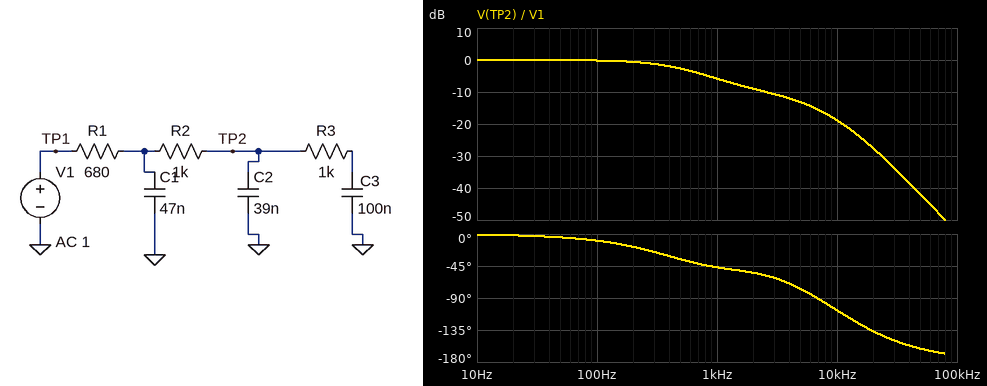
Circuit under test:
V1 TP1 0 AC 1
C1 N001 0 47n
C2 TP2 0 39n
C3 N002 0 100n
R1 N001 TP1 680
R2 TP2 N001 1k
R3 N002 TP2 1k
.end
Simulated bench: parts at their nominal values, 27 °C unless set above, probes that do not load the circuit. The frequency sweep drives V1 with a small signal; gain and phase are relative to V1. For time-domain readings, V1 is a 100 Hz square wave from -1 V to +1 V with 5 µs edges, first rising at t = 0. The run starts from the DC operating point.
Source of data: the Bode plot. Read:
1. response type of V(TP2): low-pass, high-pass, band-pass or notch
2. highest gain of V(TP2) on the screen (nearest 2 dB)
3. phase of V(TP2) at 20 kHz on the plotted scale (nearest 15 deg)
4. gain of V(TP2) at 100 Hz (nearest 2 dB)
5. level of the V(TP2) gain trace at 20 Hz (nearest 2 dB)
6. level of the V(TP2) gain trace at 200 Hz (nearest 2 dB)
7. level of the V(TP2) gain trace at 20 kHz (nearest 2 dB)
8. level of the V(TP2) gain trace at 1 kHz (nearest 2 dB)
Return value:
low-pass
0 dB
-135 deg
0 dB
0 dB
0 dB
-28 dB
-6 dB
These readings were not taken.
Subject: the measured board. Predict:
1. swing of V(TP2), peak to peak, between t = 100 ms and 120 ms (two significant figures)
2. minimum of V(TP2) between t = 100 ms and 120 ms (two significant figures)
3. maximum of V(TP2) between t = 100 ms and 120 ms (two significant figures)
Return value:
2.0 V
-1.0 V
1.0 V
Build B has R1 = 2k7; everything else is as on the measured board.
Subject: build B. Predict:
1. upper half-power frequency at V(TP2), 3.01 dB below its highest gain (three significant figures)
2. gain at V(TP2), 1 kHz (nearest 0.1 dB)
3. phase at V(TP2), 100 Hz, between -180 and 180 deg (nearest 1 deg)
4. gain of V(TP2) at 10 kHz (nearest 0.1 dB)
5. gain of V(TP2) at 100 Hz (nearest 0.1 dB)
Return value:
239 Hz
-11.8 dB
-22 deg
-29.6 dB
-0.7 dB
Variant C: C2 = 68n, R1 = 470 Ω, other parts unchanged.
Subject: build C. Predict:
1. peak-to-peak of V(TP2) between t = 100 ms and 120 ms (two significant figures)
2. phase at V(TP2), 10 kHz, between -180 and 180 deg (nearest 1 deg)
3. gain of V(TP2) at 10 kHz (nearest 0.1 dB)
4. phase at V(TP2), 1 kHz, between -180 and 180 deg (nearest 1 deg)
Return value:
2.0 V
-112 deg
-20.0 dB
-49 deg
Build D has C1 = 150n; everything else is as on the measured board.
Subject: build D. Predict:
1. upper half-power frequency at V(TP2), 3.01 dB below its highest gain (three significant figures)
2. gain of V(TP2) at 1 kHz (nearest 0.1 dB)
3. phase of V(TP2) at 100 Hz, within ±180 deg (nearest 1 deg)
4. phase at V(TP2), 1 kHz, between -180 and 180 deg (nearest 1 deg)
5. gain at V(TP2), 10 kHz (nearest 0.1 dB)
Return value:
473 Hz
-7.0 dB
-12 deg
-63 deg
-26.9 dB
